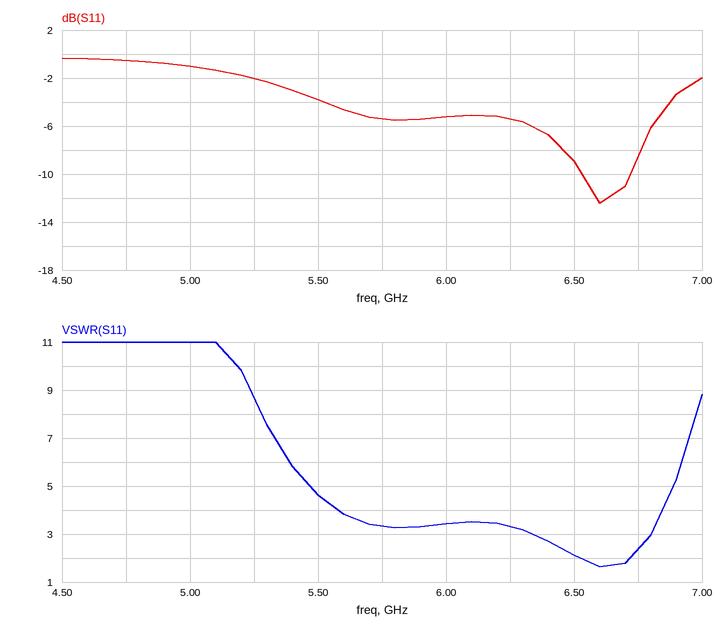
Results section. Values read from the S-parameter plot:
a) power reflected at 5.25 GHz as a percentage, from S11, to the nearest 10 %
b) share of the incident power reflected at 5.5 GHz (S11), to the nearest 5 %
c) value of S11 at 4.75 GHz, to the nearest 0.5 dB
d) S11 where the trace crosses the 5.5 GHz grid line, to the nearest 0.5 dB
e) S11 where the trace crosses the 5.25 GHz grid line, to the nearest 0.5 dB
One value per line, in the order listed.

60 %
40 %
-0.5 dB
-4.0 dB
-2.0 dB
